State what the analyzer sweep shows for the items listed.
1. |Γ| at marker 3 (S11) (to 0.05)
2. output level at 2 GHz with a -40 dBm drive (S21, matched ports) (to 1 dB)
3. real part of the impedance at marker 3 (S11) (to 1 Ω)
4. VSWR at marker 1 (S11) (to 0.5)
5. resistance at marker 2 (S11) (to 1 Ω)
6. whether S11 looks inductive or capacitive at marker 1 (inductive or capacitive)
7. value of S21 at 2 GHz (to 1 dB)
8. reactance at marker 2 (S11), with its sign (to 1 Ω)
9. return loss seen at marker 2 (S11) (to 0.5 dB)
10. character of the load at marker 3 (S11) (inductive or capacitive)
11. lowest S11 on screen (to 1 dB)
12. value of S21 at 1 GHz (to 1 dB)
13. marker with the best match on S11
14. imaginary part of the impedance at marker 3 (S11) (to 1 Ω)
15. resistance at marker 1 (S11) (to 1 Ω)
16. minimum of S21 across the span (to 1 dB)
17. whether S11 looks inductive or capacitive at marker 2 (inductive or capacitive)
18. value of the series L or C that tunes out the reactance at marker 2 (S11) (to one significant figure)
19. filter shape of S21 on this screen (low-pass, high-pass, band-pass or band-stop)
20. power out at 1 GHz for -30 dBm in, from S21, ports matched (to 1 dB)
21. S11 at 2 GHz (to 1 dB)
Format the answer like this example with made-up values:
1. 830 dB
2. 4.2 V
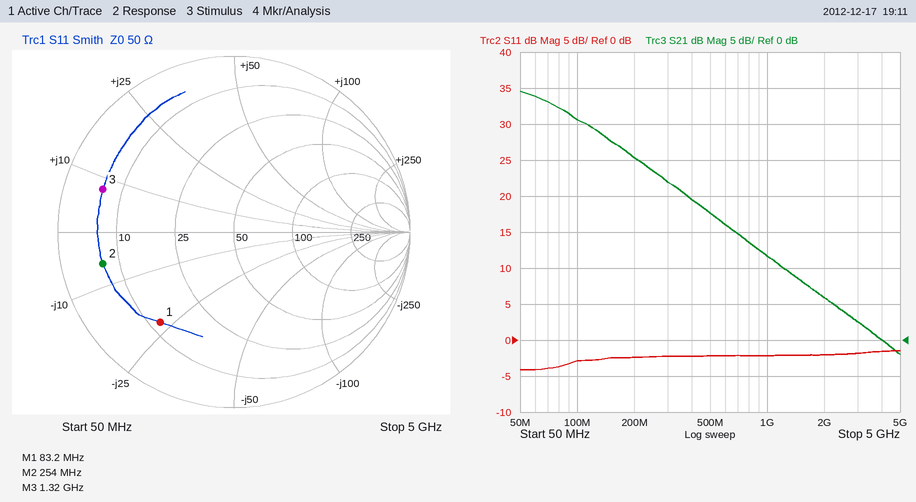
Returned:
1. 0.80
2. -34 dBm
3. 6 Ω
4. 5.0
5. 7 Ω
6. capacitive
7. 6 dB
8. -6 Ω
9. 2.5 dB
10. inductive
11. -4 dB
12. 12 dB
13. marker 1
14. +8 Ω
15. 12 Ω
16. -2 dB
17. capacitive
18. 4 nH
19. low-pass
20. -18 dBm
21. -2 dB
